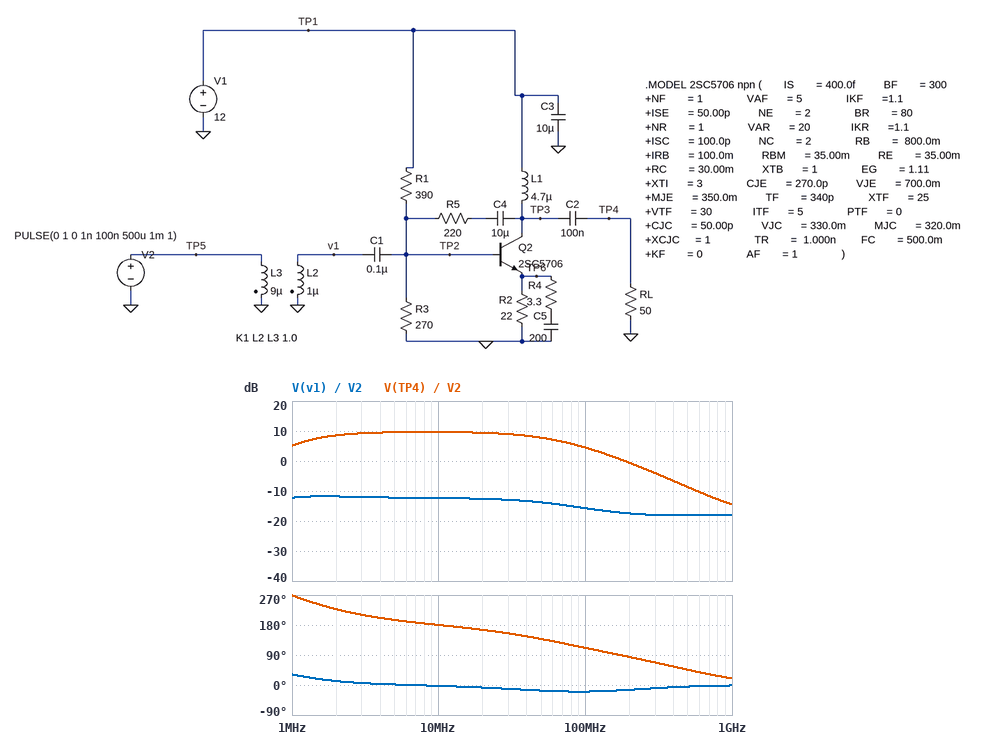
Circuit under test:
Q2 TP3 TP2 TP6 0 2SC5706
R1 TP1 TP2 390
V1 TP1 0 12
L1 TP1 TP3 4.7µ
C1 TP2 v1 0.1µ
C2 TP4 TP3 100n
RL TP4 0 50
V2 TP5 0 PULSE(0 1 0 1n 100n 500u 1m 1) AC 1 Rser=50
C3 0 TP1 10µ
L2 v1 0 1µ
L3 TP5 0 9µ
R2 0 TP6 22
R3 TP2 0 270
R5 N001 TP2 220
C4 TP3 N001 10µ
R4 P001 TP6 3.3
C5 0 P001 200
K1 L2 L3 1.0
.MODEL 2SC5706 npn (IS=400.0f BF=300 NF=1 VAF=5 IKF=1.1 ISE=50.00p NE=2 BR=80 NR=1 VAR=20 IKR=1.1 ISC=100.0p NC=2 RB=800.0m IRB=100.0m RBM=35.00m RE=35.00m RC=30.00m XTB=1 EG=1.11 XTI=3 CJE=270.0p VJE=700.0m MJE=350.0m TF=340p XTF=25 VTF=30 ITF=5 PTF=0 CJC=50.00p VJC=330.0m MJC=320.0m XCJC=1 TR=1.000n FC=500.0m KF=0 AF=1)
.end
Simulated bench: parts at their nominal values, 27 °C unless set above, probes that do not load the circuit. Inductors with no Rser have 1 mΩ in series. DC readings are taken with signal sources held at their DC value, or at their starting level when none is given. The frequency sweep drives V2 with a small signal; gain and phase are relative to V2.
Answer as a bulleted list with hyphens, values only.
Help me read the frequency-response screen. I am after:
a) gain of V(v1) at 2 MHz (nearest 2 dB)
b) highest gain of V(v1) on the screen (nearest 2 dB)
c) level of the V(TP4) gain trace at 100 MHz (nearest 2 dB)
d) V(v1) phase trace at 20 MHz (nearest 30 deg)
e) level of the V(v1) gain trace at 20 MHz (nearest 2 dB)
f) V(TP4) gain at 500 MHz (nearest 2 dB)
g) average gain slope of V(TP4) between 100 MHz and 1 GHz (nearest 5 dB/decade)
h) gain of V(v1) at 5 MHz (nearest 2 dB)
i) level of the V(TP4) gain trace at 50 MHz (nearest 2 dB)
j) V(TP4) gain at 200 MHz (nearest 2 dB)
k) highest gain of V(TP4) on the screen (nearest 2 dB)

- -12 dB
- -12 dB
- 4 dB
- 0 deg
- -12 dB
- -8 dB
- -20 dB/decade
- -12 dB
- 8 dB
- 0 dB
- 10 dB
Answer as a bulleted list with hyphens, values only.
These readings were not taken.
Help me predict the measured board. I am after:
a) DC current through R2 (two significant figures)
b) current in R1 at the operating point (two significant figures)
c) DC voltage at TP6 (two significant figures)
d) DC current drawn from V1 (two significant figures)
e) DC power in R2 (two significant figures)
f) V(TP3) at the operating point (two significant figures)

- 190 mA
- 18 mA
- 4.2 V
- 210 mA
- 790 mW
- 12 V
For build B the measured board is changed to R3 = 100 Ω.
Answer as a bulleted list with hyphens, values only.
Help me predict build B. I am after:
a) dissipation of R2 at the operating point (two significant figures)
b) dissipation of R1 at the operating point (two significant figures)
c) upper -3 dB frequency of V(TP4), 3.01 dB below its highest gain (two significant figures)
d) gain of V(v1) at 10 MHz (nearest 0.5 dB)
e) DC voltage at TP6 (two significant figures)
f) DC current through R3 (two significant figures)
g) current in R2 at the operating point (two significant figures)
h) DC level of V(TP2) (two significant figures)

- 150 mW
- 230 mW
- 70 MHz
- -12.5 dB
- 1.8 V
- 24 mA
- 81 mA
- 2.4 V
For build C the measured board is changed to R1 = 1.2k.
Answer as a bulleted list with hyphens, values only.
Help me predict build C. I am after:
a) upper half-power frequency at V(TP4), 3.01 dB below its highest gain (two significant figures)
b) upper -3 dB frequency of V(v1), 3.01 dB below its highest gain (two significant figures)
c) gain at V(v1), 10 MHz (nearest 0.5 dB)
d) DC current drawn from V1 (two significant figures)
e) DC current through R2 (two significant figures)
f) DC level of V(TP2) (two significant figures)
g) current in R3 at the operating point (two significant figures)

- 69 MHz
- 77 MHz
- -12.0 dB
- 78 mA
- 70 mA
- 2.2 V
- 8.1 mA
